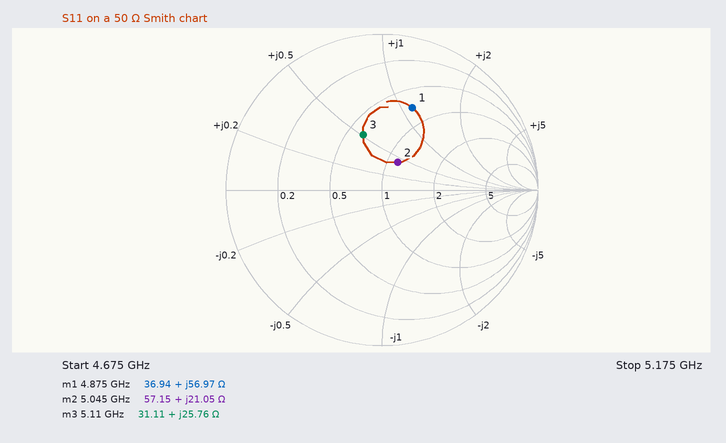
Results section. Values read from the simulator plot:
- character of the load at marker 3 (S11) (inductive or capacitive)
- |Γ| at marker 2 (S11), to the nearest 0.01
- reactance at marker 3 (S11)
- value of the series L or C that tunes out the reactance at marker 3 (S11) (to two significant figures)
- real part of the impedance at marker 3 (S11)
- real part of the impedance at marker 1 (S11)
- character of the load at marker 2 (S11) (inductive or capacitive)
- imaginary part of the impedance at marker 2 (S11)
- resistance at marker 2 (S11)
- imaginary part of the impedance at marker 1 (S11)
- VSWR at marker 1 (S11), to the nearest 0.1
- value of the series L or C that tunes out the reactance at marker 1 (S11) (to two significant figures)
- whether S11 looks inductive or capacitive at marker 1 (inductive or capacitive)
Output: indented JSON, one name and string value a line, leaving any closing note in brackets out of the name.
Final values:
{
  "character of the load at marker 3 (S11)": "inductive",
  "|Γ| at marker 2 (S11), to the nearest 0.01": "0.20",
  "reactance at marker 3": "+25.76 Ω",
  "value of the series L or C that tunes out the reactance at marker 3 (S11)": "1.2 pF",
  "real part of the impedance at marker 3": "31.11 Ω",
  "real part of the impedance at marker 1": "36.94 Ω",
  "character of the load at marker 2 (S11)": "inductive",
  "imaginary part of the impedance at marker 2": "+21.05 Ω",
  "resistance at marker 2": "57.15 Ω",
  "imaginary part of the impedance at marker 1": "+56.97 Ω",
  "VSWR at marker 1 (S11), to the nearest 0.1": "3.6",
  "value of the series L or C that tunes out the reactance at marker 1 (S11)": "570 fF",
  "whether S11 looks inductive or capacitive at marker 1": "inductive"
}
